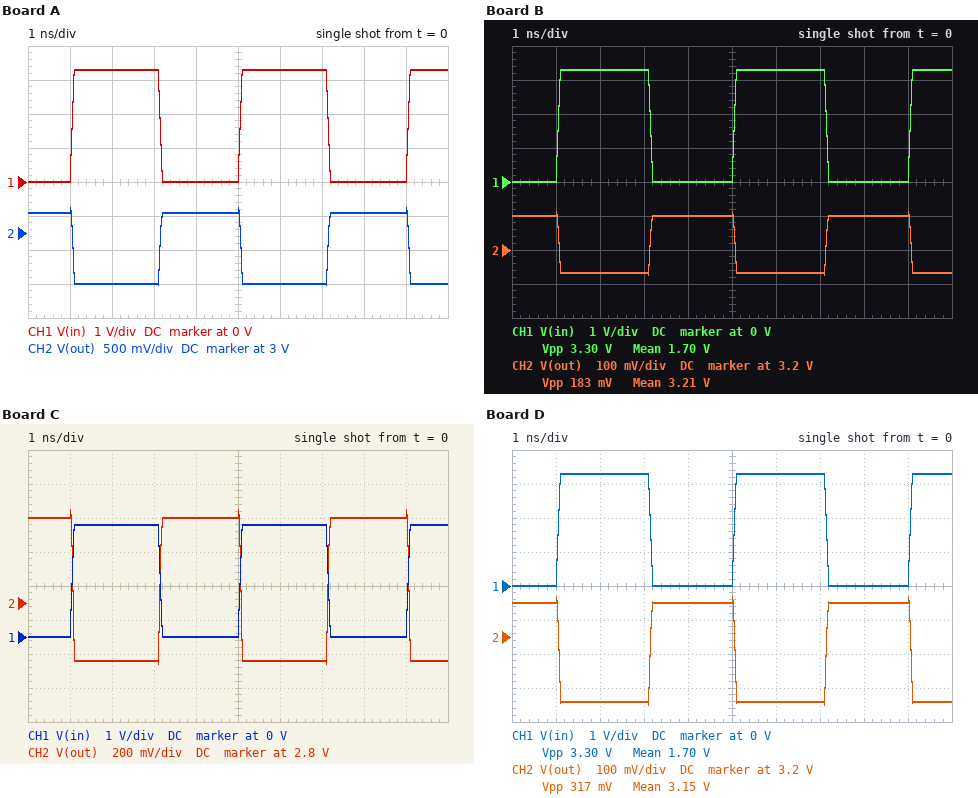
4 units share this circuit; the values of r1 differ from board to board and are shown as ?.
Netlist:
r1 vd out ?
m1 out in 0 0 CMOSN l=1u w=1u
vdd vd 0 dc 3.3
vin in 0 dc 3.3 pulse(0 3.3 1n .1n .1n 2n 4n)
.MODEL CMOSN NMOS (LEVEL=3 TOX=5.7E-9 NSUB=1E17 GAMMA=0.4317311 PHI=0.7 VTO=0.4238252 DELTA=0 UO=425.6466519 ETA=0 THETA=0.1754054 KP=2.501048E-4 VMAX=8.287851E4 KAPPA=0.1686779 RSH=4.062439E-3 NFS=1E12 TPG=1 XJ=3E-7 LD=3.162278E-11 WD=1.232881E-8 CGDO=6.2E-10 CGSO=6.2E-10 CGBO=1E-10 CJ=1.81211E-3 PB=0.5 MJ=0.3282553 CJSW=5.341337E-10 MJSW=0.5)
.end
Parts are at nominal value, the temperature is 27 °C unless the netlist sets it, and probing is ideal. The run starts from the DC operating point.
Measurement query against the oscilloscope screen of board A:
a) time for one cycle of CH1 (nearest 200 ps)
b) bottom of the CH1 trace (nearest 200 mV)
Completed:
4.0 ns
0 V
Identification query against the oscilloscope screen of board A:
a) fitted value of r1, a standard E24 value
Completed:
3 kΩ
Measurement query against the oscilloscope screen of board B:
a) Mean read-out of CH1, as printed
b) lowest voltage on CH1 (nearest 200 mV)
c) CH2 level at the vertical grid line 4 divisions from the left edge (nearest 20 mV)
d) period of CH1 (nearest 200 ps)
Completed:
1.70 V
0 V
3.30 V
4.0 ns
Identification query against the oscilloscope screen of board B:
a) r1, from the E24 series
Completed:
470 Ω
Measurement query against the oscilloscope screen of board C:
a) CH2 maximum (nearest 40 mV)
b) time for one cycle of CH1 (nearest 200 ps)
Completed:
3.36 V
4.0 ns
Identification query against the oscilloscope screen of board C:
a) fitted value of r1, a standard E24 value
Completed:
2.4 kΩ
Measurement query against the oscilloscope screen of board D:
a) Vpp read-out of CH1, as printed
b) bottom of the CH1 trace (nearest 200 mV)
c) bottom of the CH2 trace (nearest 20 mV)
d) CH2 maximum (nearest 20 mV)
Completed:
3.30 V
0 V
3.00 V
3.32 V
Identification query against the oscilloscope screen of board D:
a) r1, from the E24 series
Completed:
820 Ω
